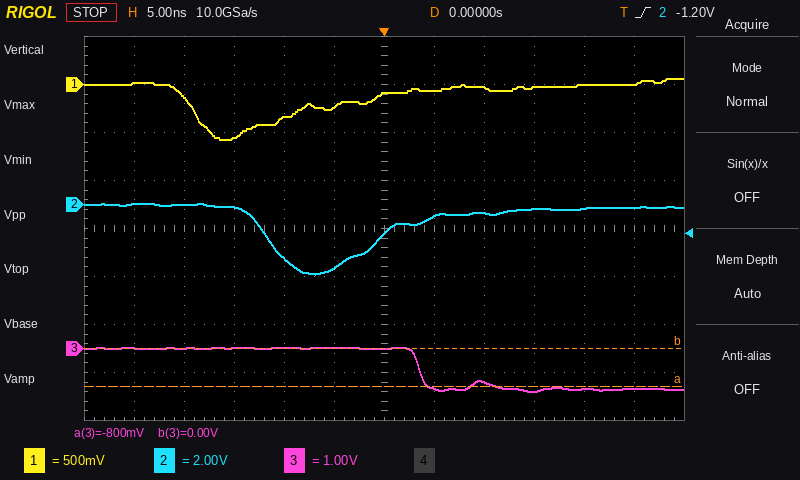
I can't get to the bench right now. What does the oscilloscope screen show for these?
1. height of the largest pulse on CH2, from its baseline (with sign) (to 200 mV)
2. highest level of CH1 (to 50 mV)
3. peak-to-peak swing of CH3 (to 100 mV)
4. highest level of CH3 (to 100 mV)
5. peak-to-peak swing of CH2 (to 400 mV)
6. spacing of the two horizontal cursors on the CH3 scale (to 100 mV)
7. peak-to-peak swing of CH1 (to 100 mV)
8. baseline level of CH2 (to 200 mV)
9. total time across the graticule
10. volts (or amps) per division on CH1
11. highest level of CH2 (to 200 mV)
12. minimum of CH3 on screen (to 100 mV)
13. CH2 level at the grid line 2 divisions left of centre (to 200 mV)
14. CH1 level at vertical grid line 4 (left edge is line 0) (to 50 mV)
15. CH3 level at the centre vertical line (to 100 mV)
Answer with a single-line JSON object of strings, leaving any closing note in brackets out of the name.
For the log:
{"height of the largest pulse on CH2, from its baseline (with sign)": "-2.8 V", "highest level of CH1": "50 mV", "peak-to-peak swing of CH3": "900 mV", "highest level of CH3": "0.0 V", "peak-to-peak swing of CH2": "2.8 V", "spacing of the two horizontal cursors on the CH3 scale": "800 mV", "peak-to-peak swing of CH1": "600 mV", "baseline level of CH2": "-200 mV", "total time across the graticule": "60 ns", "volts (or amps) per division on CH1": "500 mV", "highest level of CH2": "0.0 V", "minimum of CH3 on screen": "-900 mV", "CH2 level at the grid line 2 divisions left of centre": "-2.2 V", "CH1 level at vertical grid line 4 (left edge is line 0)": "-350 mV", "CH3 level at the centre vertical line": "0.0 V"}
